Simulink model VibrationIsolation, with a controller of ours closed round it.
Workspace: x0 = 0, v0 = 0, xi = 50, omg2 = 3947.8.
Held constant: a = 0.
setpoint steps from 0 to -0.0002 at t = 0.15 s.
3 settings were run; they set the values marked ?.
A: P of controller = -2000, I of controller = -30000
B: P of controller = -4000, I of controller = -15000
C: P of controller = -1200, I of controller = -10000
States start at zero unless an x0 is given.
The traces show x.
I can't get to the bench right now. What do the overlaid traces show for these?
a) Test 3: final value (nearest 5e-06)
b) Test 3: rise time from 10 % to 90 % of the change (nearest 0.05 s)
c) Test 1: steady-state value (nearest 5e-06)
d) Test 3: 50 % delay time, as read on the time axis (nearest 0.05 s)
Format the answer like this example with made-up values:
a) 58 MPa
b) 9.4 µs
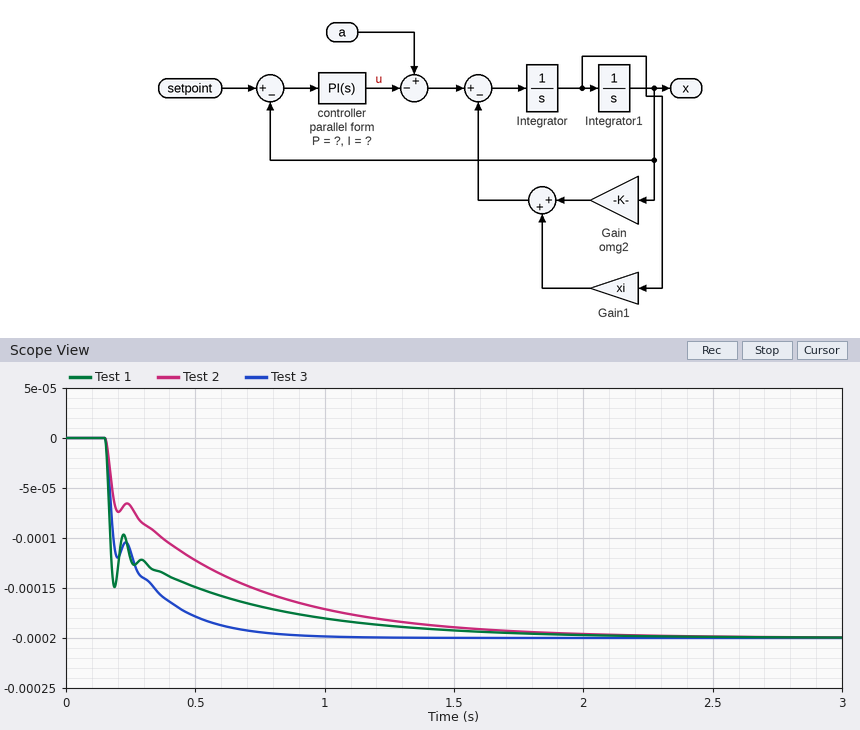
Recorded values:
a) -0.000200
b) 0.35 s
c) -0.000200
d) 0.20 s
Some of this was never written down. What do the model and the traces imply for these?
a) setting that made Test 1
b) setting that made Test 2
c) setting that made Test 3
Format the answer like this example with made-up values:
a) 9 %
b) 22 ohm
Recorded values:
a) B
b) C
c) A
